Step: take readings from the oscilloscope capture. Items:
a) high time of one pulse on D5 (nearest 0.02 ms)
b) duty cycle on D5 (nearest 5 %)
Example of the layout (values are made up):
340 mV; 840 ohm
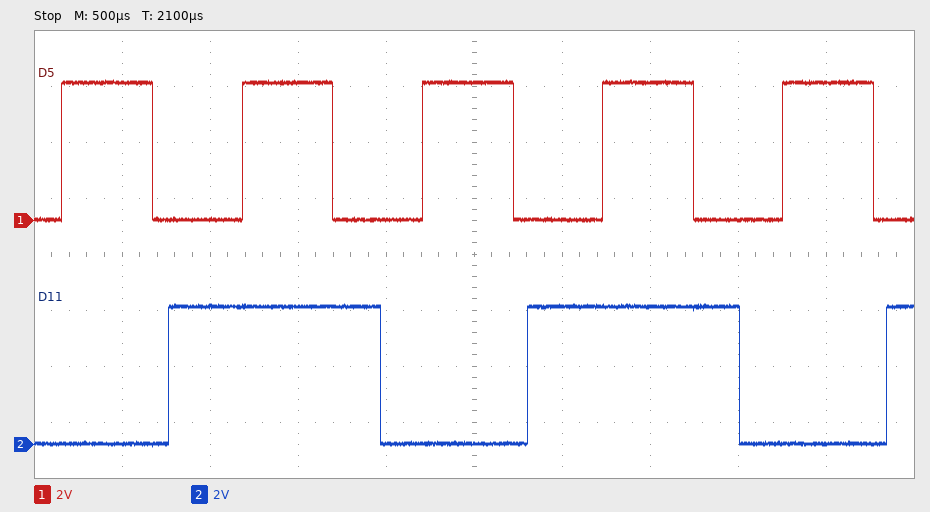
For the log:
0.52 ms; 50 %
